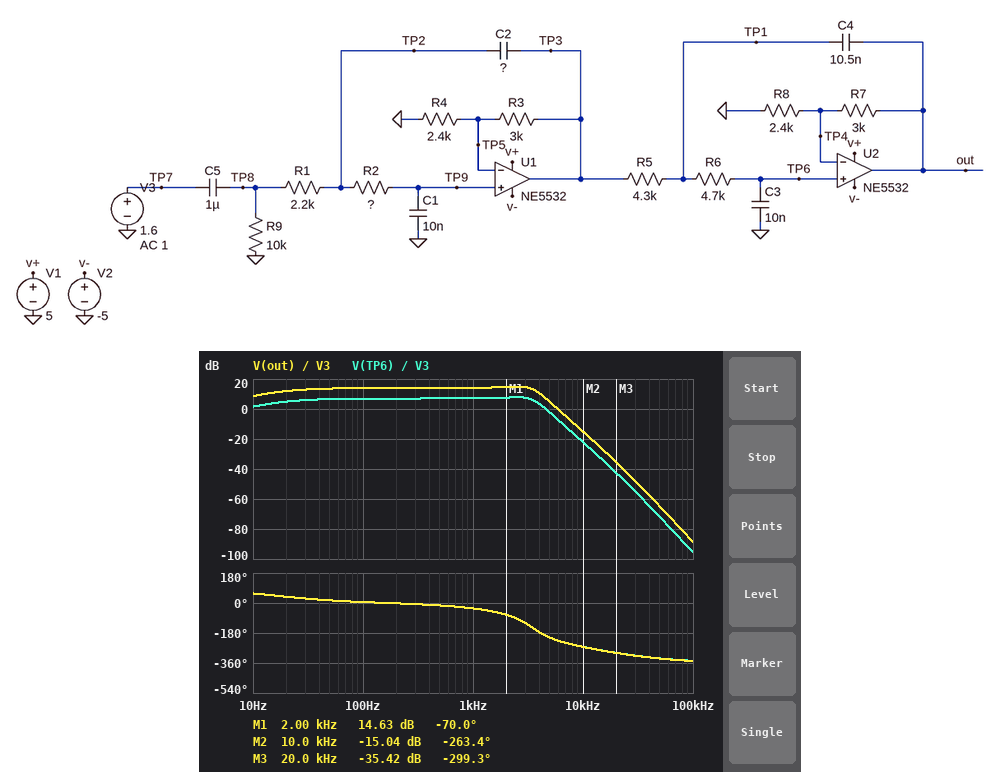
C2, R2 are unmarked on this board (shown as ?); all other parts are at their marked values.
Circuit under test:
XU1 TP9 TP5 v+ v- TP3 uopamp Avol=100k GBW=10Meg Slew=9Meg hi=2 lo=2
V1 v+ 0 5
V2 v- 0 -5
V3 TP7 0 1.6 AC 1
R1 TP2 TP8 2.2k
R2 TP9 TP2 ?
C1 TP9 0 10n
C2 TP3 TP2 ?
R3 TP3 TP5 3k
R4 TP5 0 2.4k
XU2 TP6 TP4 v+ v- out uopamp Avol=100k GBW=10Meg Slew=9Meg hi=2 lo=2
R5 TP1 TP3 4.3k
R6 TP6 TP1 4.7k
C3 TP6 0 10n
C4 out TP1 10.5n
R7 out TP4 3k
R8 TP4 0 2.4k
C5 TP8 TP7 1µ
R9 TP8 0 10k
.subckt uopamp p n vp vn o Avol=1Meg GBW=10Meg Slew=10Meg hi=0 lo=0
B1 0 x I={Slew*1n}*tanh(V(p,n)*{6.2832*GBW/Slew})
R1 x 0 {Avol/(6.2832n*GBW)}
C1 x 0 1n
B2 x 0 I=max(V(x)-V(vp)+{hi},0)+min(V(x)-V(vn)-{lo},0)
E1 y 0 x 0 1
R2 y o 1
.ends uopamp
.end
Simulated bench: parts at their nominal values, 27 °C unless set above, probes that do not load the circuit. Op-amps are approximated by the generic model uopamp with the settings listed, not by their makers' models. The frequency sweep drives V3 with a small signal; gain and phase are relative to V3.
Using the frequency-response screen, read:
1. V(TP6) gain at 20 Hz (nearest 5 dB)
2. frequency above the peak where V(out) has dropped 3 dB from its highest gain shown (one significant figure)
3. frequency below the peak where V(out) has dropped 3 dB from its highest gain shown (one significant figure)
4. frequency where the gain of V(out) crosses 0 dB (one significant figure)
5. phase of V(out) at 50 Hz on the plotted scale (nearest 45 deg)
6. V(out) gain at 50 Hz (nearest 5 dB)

5 dB
4 kHz
20 Hz
6 kHz
0 deg
15 dB
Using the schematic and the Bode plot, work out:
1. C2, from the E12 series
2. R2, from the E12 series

3.9 nF
4.7 kΩ
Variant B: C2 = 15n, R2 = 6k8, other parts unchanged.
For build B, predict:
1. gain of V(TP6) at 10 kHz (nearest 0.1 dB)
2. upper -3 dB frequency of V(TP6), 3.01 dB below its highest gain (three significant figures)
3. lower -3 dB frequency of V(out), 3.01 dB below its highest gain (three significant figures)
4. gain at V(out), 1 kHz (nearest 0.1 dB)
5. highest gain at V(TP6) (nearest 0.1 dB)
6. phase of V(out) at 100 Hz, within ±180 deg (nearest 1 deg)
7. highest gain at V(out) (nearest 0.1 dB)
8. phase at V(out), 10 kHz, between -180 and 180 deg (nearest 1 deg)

-29.2 dB
3.63 kHz
1.05 kHz
15.0 dB
11.1 dB
6 deg
18.1 dB
37 deg
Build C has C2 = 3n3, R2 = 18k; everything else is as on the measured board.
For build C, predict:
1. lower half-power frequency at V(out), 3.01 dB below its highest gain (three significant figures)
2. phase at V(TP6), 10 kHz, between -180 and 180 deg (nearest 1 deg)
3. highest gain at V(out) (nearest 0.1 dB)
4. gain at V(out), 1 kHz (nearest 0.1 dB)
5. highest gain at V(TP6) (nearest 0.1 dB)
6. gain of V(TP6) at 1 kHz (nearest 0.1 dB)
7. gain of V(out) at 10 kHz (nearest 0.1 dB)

15.3 Hz
87 deg
13.9 dB
10.8 dB
6.8 dB
3.8 dB
-25.8 dB
